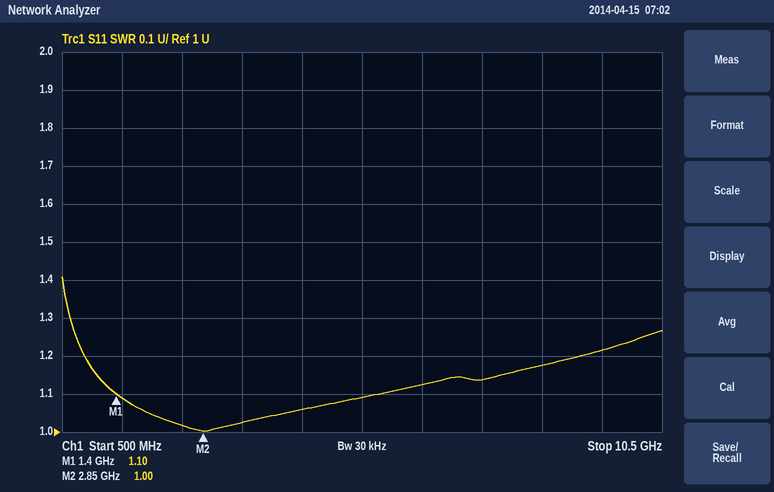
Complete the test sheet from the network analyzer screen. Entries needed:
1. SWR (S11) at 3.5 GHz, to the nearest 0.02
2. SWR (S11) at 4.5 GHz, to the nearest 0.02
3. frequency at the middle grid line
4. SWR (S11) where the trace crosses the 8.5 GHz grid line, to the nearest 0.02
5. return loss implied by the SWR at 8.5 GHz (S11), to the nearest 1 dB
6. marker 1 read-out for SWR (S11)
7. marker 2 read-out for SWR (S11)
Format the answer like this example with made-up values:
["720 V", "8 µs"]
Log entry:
["1.02", "1.06", "5.5 GHz", "1.18", "22 dB", "1.10", "1.00"]
